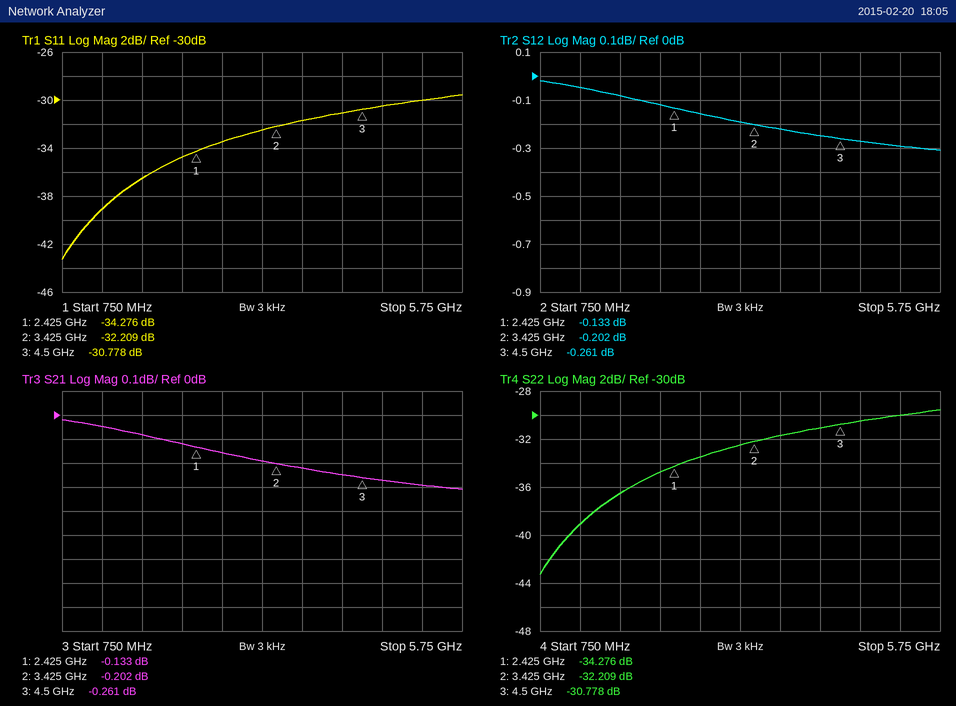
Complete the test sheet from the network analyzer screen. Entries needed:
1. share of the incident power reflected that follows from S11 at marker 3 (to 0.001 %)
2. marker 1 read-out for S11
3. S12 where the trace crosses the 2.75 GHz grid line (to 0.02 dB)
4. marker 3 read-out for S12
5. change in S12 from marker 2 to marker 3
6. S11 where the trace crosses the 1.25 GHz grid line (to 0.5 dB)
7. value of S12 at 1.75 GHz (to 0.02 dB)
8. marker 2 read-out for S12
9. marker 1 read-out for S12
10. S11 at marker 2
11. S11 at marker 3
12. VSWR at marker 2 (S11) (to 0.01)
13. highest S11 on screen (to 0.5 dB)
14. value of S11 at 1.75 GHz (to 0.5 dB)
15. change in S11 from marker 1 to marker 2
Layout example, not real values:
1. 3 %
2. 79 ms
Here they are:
1. 0.084 %
2. -34.276 dB
3. -0.16 dB
4. -0.261 dB
5. -0.059 dB
6. -39.0 dB
7. -0.08 dB
8. -0.202 dB
9. -0.133 dB
10. -32.209 dB
11. -30.778 dB
12. 1.05
13. -29.5 dB
14. -36.5 dB
15. 2.067 dB
